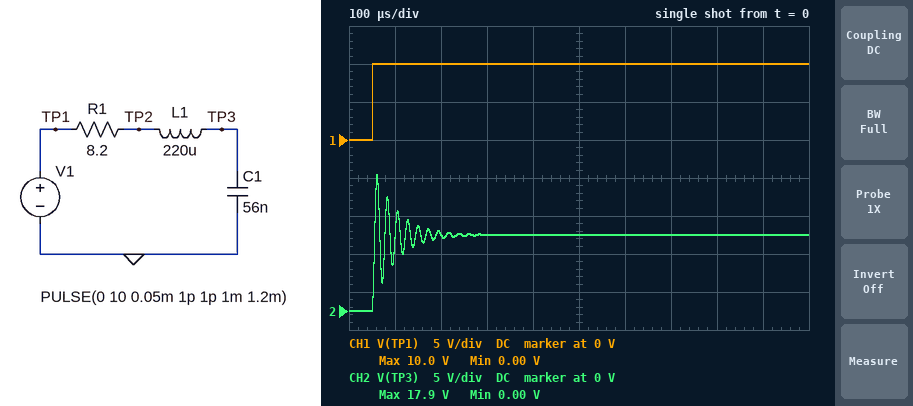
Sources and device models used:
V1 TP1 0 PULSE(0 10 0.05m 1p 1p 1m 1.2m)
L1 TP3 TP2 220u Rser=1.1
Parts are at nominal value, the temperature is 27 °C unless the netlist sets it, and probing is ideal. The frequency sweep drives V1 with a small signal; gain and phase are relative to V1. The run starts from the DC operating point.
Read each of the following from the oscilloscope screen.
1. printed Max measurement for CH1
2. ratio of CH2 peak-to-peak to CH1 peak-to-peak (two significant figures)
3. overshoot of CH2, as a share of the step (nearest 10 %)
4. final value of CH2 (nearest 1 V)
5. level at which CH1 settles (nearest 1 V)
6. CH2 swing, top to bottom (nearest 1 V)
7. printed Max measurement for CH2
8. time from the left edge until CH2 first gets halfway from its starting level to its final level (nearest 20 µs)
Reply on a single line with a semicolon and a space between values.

10.0 V; 1.8; 80 %; 10 V; 10 V; 18 V; 17.9 V; 60 µs
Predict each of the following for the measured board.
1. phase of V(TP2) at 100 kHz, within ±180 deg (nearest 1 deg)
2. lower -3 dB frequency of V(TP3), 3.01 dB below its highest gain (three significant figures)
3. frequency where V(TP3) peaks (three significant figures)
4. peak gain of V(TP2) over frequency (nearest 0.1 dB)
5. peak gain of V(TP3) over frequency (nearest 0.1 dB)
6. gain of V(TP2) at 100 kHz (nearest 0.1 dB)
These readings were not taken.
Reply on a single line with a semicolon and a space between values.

4 deg; 41.6 kHz; 45.1 kHz; 0 dB; 16.6 dB; 0 dB
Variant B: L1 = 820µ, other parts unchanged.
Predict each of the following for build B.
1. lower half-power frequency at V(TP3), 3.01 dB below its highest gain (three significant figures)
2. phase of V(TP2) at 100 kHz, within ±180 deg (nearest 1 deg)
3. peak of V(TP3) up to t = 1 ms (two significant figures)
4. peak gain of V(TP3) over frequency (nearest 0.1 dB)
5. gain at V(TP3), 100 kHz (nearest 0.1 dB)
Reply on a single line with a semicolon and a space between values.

22.5 kHz; 1 deg; 19 V; 22.3 dB; -24.7 dB
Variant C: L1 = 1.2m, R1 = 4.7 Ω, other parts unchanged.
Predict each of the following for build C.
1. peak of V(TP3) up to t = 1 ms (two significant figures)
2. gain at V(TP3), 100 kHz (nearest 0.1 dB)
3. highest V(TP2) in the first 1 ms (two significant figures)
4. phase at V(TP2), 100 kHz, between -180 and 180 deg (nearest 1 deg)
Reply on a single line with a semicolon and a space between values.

19 V; -28.1 dB; 10 V; 0 deg
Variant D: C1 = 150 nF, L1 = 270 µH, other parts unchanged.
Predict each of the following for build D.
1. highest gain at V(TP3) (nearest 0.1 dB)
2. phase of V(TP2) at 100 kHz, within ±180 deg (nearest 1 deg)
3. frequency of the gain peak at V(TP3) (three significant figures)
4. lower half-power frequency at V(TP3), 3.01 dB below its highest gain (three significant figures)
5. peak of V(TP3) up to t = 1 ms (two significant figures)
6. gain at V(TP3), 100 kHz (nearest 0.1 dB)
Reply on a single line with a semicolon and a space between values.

13.2 dB; 3 deg; 24.7 kHz; 21.8 kHz; 17 V; -23.5 dB
